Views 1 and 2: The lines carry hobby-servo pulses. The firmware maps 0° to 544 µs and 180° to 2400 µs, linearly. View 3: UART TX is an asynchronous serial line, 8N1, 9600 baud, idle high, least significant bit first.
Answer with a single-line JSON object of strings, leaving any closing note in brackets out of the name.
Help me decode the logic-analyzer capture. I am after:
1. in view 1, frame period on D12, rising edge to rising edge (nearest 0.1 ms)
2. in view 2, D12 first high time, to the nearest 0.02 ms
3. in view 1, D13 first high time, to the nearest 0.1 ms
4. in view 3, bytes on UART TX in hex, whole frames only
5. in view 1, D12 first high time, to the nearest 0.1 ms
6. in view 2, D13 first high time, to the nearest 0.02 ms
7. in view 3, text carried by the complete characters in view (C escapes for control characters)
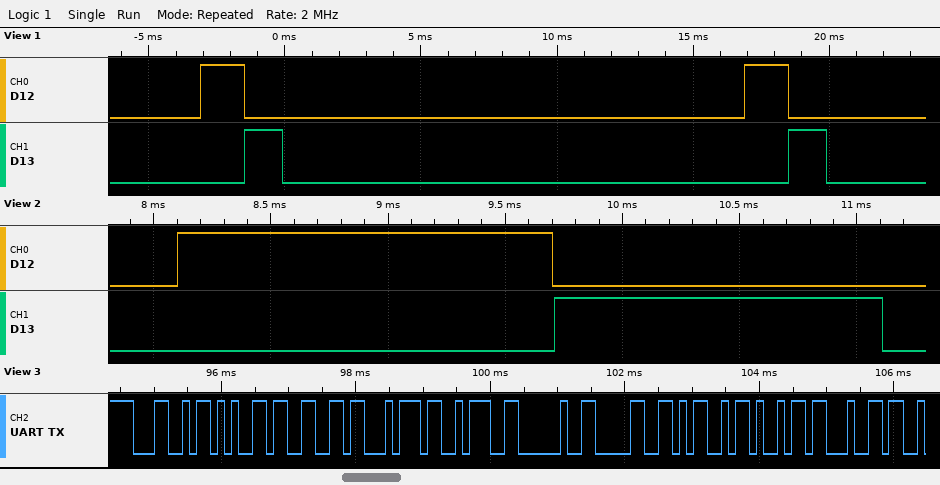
{"in view 1, frame period on D12, rising edge to rising edge": "20.0 ms", "in view 2, D12 first high time, to the nearest 0.02 ms": "1.60 ms", "in view 1, D13 first high time, to the nearest 0.1 ms": "1.4 ms", "in view 3, bytes on UART TX in hex, whole frames only": "4C 65 66 74 3A 20 30 4D 69 64", "in view 1, D12 first high time, to the nearest 0.1 ms": "1.6 ms", "in view 2, D13 first high time, to the nearest 0.02 ms": "1.40 ms", "in view 3, text carried by the complete characters in view": "\"Left: 0Mid\""}
